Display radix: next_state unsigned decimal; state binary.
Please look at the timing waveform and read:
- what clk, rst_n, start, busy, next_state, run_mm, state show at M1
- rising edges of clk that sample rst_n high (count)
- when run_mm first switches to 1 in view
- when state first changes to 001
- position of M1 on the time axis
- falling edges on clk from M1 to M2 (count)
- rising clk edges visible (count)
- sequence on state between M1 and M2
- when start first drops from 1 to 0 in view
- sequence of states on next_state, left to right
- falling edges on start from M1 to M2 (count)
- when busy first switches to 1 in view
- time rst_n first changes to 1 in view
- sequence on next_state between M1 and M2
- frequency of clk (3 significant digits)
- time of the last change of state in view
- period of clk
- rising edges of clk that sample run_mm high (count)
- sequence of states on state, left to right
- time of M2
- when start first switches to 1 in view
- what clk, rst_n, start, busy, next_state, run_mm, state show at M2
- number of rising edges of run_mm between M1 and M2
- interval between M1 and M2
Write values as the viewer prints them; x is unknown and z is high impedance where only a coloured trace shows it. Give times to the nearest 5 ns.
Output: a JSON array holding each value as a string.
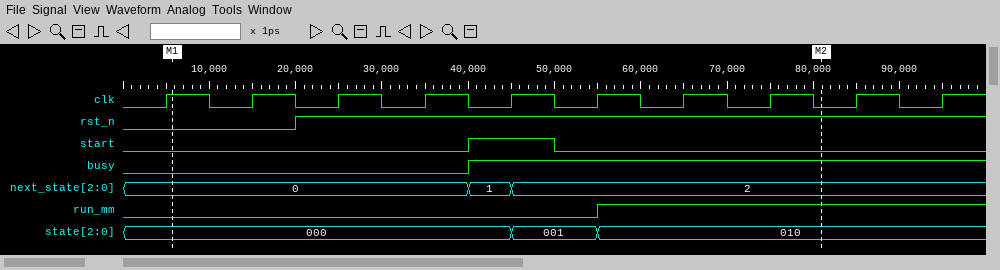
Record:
["clk=1, rst_n=0, start=0, busy=0, next_state=0, run_mm=0, state=000", "8", "55 ns", "45 ns", "5 ns", "8", "10", "000, 001, 010", "50 ns", "0, 1, 2", "1", "40 ns", "20 ns", "0, 1, 2", "100 MHz", "55 ns", "10 ns", "4", "000, 001, 010", "80 ns", "40 ns", "clk=0, rst_n=1, start=0, busy=1, next_state=2, run_mm=1, state=010", "1", "75 ns"]
